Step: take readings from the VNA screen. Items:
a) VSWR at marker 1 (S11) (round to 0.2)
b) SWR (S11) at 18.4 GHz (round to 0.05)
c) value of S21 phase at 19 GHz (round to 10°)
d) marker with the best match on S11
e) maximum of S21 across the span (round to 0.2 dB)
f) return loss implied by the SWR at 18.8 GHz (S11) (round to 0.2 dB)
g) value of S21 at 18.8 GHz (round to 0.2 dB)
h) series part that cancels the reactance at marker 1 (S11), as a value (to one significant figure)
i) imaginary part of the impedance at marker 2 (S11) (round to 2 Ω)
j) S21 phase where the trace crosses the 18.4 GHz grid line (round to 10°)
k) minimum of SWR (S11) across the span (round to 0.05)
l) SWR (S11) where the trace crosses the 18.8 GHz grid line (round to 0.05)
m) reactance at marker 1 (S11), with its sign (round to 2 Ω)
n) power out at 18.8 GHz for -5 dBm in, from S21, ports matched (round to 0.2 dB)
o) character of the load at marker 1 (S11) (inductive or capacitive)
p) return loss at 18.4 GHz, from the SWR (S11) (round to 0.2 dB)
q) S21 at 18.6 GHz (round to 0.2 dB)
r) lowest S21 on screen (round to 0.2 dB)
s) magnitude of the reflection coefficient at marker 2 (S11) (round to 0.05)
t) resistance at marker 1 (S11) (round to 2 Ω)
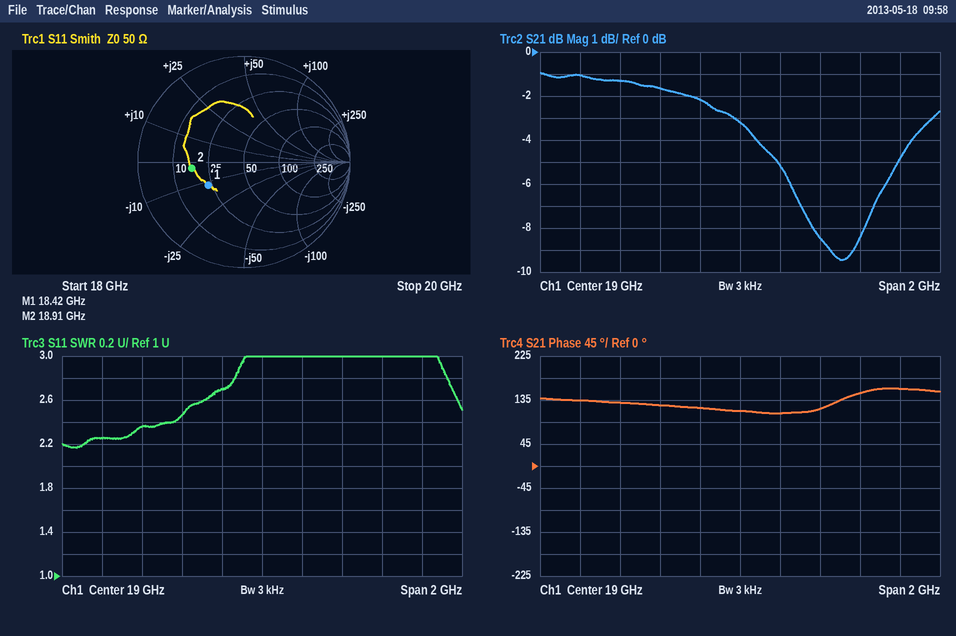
2.4
2.35
110°
marker 1
-1.0 dB
6.8 dB
-2.2 dB
100 pH
-2 Ω
130°
2.15
2.70
-12 Ω
-7.2 dBm
capacitive
7.8 dB
-1.6 dB
-9.4 dB
0.50
22 Ω
